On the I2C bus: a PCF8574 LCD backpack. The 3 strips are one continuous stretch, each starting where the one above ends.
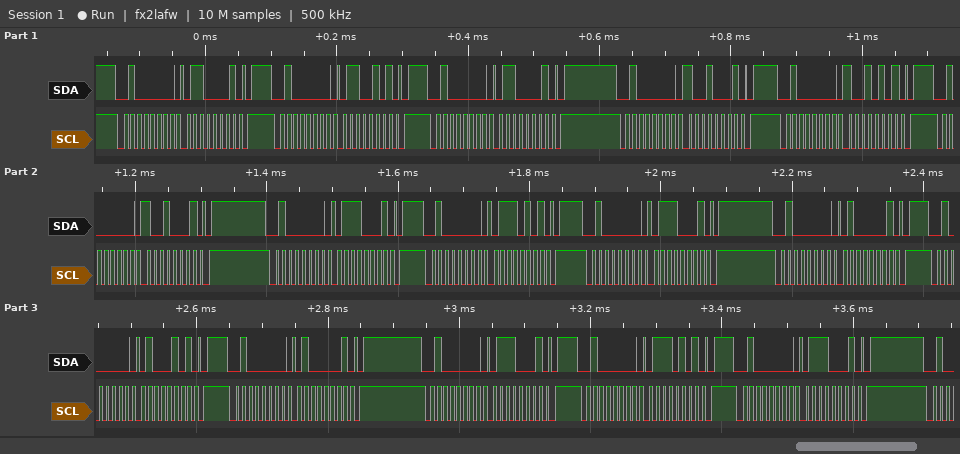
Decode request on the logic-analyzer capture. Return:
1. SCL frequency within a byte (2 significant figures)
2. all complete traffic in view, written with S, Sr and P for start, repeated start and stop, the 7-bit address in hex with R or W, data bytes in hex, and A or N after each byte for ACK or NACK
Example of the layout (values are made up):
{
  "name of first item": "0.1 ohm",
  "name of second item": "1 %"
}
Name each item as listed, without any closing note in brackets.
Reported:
{
  "SCL frequency within a byte": "100 kHz",
  "all complete traffic in view, written with S, Sr and P for start, repeated start and stop, the 7-bit address in hex with R or W, data bytes in hex, and A or N after each byte for ACK or NACK": "S 20W A 61 A P S 20W A 65 A P S 20W A 61 A P S 20W A 91 A P S 20W A 95 A P S 20W A 91 A P S 20W A 71 A P S 20W A 75 A P S 20W A 71 A P S 20W A 41 A P S 20W A 45 A P S 20W A 41 A P S 20W A 71 A P S 20W A 75 A P S 20W A 71 A P"
}
